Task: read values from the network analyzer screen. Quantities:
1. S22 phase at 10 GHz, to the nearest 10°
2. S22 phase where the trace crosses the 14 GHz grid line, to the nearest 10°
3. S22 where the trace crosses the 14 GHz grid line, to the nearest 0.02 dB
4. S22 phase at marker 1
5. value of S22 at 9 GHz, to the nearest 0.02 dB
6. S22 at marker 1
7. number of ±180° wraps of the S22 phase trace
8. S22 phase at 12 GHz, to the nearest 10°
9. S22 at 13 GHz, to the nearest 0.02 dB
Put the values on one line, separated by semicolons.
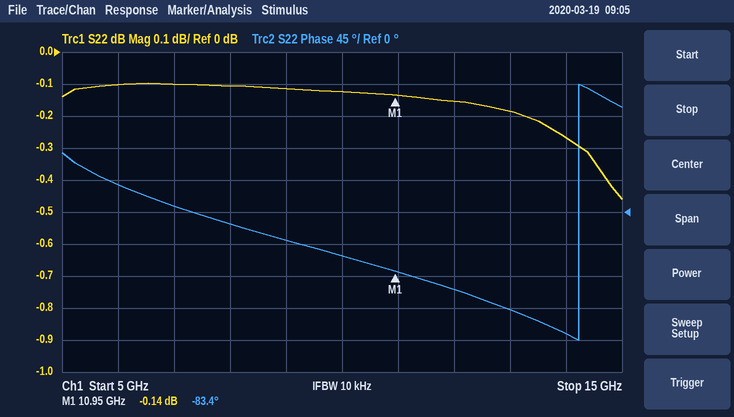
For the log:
-60°; -170°; -0.26 dB; -83.4°; -0.12 dB; -0.14 dB; 1; -110°; -0.18 dB
